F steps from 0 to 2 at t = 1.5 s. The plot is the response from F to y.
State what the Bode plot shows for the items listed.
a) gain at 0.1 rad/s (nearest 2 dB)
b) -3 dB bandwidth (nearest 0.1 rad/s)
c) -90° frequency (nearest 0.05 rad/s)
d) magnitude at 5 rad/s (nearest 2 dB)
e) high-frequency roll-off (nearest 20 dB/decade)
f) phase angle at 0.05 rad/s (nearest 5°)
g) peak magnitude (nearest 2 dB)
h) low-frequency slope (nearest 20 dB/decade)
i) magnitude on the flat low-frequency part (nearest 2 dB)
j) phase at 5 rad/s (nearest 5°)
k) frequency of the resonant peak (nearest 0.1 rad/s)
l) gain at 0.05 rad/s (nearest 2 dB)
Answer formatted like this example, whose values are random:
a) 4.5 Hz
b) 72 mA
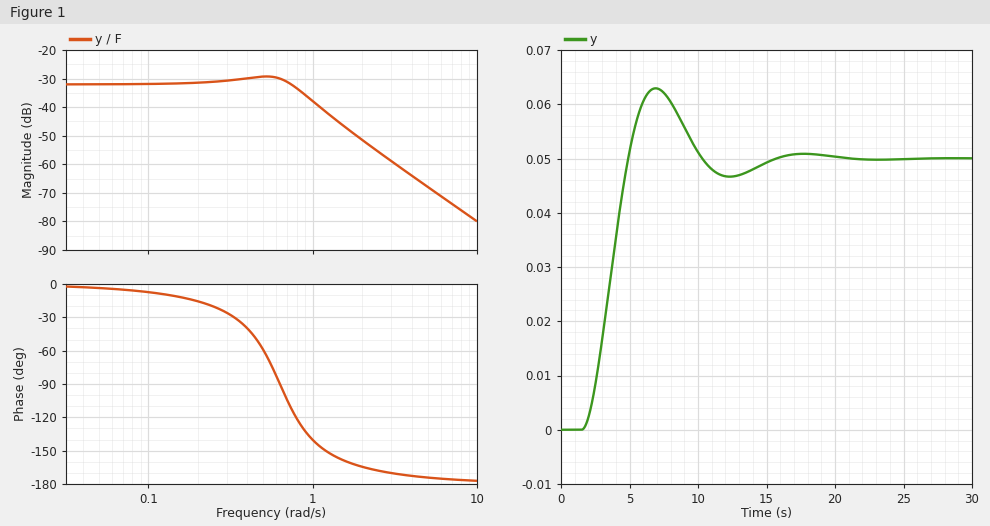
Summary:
a) -32 dB
b) 0.9 rad/s
c) 0.65 rad/s
d) -68 dB
e) -40 dB/decade
f) -5°
g) -30 dB
h) 0 dB/decade
i) -32 dB
j) -175°
k) 0.5 rad/s
l) -32 dB
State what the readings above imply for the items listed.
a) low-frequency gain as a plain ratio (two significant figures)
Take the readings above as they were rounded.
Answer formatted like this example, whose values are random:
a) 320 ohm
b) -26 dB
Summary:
a) 0.025
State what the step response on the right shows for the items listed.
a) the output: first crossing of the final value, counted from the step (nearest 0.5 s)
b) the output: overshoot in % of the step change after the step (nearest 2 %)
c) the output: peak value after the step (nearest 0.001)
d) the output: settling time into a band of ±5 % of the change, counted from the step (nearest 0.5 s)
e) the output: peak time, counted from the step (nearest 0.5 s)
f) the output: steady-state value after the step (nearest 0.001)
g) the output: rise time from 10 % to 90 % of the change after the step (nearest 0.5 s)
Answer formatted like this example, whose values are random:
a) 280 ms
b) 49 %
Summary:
a) 3.5 s
b) 26 %
c) 0.063
d) 12.0 s
e) 5.5 s
f) 0.050
g) 2.5 s
